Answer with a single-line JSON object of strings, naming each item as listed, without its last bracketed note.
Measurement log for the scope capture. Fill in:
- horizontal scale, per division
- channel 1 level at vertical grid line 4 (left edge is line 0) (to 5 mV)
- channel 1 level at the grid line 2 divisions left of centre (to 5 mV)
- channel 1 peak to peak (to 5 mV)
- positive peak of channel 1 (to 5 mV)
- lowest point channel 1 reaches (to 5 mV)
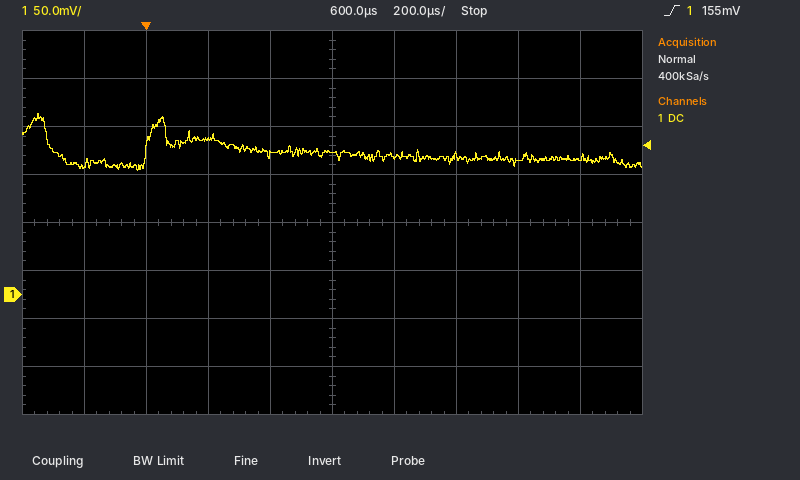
{"horizontal scale, per division": "200 µs", "channel 1 level at vertical grid line 4 (left edge is line 0)": "145 mV", "channel 1 level at the grid line 2 divisions left of centre": "160 mV", "channel 1 peak to peak": "60 mV", "positive peak of channel 1": "190 mV", "lowest point channel 1 reaches": "130 mV"}
